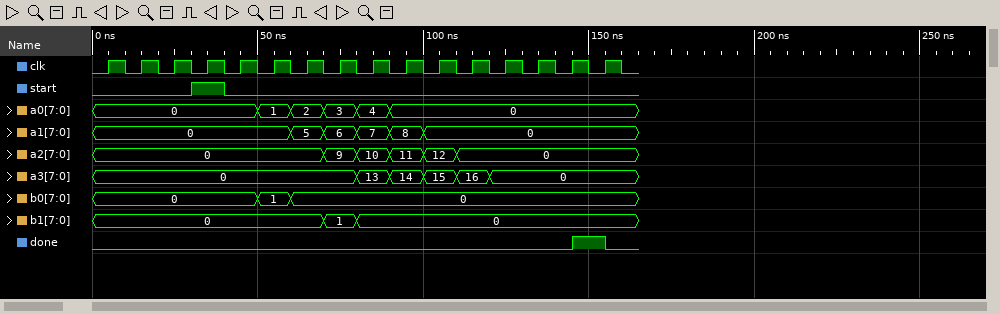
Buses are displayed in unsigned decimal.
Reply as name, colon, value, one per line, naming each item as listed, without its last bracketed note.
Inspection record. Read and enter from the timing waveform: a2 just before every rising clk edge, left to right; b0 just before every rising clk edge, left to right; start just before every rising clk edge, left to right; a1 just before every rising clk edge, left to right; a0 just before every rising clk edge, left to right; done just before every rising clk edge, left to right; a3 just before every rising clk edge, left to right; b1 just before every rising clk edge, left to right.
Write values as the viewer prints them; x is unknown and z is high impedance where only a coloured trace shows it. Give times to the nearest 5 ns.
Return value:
a2 just before every rising clk edge, left to right: 0, 0, 0, 0, 0, 0, 0, 9, 10, 11, 12, 0, 0, 0, 0, 0
b0 just before every rising clk edge, left to right: 0, 0, 0, 0, 0, 1, 0, 0, 0, 0, 0, 0, 0, 0, 0, 0
start just before every rising clk edge, left to right: 0 0 0 1 0 0 0 0 0 0 0 0 0 0 0 0
a1 just before every rising clk edge, left to right: 0, 0, 0, 0, 0, 0, 5, 6, 7, 8, 0, 0, 0, 0, 0, 0
a0 just before every rising clk edge, left to right: 0, 0, 0, 0, 0, 1, 2, 3, 4, 0, 0, 0, 0, 0, 0, 0
done just before every rising clk edge, left to right: 0 0 0 0 0 0 0 0 0 0 0 0 0 0 0 1
a3 just before every rising clk edge, left to right: 0, 0, 0, 0, 0, 0, 0, 0, 13, 14, 15, 16, 0, 0, 0, 0
b1 just before every rising clk edge, left to right: 0, 0, 0, 0, 0, 0, 0, 1, 0, 0, 0, 0, 0, 0, 0, 0
